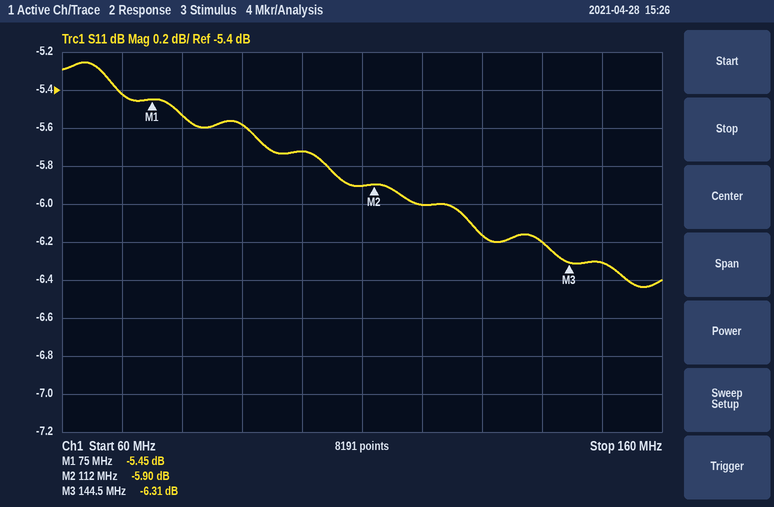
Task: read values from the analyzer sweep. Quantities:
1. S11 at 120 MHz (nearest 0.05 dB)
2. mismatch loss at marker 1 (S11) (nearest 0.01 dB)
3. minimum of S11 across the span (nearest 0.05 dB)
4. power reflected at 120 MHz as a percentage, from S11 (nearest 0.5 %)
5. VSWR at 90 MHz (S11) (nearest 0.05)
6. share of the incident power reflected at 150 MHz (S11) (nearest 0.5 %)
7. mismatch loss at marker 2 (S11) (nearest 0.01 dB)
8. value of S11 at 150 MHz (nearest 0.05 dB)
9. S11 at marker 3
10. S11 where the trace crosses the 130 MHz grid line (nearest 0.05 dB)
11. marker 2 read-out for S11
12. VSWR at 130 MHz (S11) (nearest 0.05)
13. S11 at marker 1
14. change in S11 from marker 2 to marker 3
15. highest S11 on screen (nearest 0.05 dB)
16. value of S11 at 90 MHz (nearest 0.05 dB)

-6.00 dB
1.46 dB
-6.45 dB
25.0 %
3.20
23.5 %
1.29 dB
-6.30 dB
-6.31 dB
-6.15 dB
-5.90 dB
2.95
-5.45 dB
-0.41 dB
-5.25 dB
-5.60 dB
